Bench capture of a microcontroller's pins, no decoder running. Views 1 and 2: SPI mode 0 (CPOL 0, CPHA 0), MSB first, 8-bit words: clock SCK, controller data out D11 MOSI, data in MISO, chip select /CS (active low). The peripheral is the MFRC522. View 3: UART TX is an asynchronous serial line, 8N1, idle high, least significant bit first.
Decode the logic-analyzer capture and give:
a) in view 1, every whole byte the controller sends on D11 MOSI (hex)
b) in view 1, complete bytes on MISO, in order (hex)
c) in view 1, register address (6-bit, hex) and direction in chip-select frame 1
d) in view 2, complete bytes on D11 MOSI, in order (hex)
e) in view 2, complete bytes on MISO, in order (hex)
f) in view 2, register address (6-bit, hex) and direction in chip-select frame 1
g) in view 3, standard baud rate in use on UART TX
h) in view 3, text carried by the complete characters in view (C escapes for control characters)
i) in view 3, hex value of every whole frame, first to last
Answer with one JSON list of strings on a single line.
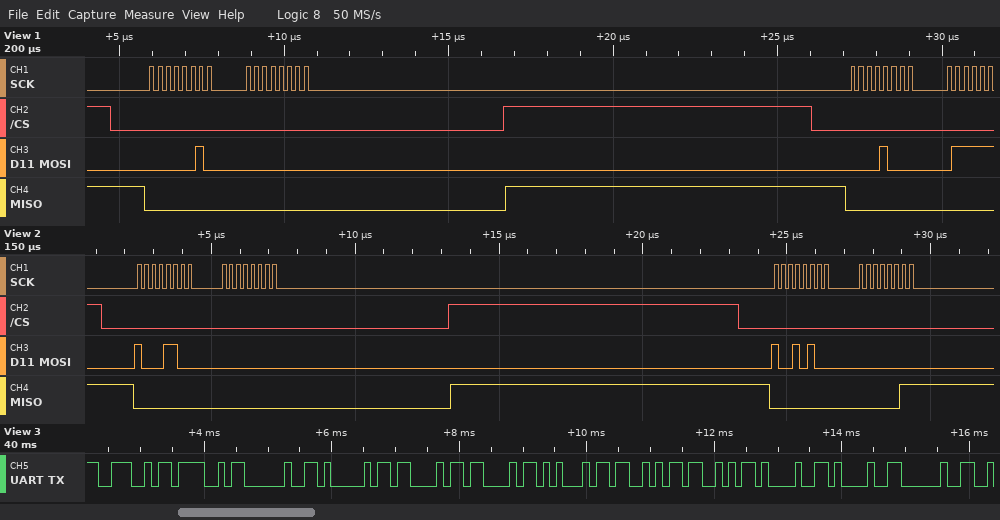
["02 00 08", "00 00 00", "0x01 write", "8C 00 94 00", "00 00 00 03", "0x06 read", "9600 baud", "\"NO ACCESS!! \"", "4E 4F 20 41 43 43 45 53 53 21 21 20"]
